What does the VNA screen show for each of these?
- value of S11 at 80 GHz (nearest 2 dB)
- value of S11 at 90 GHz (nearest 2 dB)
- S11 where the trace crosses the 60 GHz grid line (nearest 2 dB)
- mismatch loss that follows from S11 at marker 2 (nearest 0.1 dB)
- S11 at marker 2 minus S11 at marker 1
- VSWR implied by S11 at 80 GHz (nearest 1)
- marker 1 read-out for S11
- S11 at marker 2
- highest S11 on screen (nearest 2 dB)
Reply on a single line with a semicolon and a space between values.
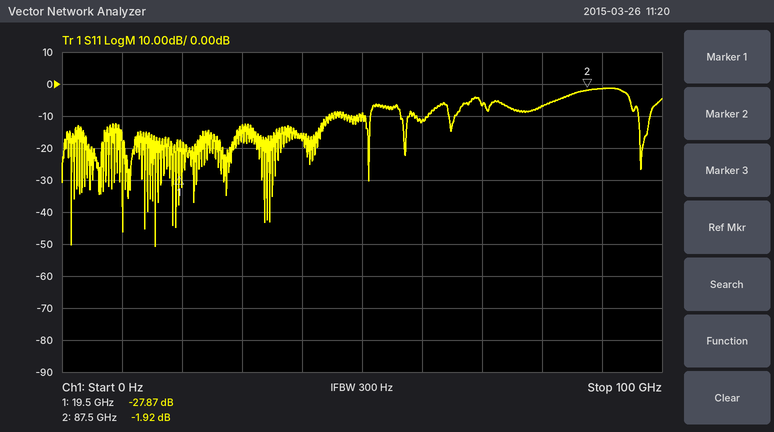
-6 dB; -2 dB; -12 dB; 4.5 dB; 25.95 dB; 3; -27.87 dB; -1.92 dB; -2 dB
